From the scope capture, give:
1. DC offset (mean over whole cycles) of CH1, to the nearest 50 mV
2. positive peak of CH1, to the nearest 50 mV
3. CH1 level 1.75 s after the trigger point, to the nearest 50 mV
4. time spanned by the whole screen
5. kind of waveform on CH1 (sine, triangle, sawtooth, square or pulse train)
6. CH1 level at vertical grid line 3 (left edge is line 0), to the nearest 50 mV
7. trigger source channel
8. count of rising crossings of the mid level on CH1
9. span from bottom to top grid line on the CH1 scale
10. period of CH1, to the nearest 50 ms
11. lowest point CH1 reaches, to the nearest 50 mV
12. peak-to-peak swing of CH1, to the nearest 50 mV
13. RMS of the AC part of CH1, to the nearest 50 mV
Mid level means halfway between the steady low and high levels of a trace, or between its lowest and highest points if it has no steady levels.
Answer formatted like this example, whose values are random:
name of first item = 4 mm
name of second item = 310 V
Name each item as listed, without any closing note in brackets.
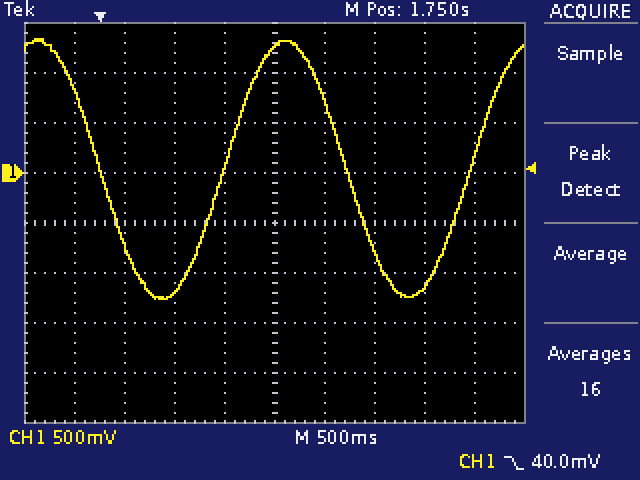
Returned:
DC offset (mean over whole cycles) of CH1, to the nearest 50 mV = 50 mV
positive peak of CH1, to the nearest 50 mV = 1.35 V
CH1 level 1.75 s after the trigger point, to the nearest 50 mV = 1.25 V
time spanned by the whole screen = 5 s
kind of waveform on CH1 = sine
CH1 level at vertical grid line 3 (left edge is line 0), to the nearest 50 mV = -1.20 V
trigger source channel = CH1
count of rising crossings of the mid level on CH1 = 2
span from bottom to top grid line on the CH1 scale = 4 V
period of CH1, to the nearest 50 ms = 2.45 s
lowest point CH1 reaches, to the nearest 50 mV = -1.25 V
peak-to-peak swing of CH1, to the nearest 50 mV = 2.60 V
RMS of the AC part of CH1, to the nearest 50 mV = 900 mV
